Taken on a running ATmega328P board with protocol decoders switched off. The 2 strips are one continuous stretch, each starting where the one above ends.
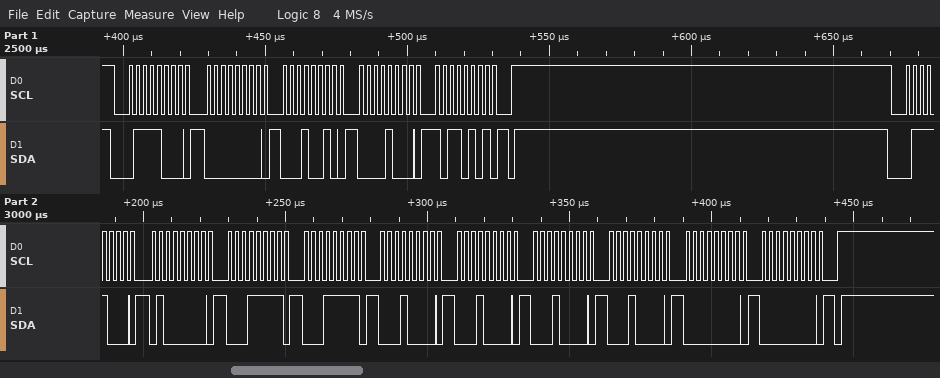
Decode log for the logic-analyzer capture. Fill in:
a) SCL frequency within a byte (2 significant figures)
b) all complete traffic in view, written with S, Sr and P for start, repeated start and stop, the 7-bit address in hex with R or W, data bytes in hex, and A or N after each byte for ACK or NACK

400 kHz
S 3CW A 00 A 12 A 08 A B5 A P S 3CW A 40 A 1F A 1F A 10 A 10 A 10 A 10 A 00 A 00 A P
